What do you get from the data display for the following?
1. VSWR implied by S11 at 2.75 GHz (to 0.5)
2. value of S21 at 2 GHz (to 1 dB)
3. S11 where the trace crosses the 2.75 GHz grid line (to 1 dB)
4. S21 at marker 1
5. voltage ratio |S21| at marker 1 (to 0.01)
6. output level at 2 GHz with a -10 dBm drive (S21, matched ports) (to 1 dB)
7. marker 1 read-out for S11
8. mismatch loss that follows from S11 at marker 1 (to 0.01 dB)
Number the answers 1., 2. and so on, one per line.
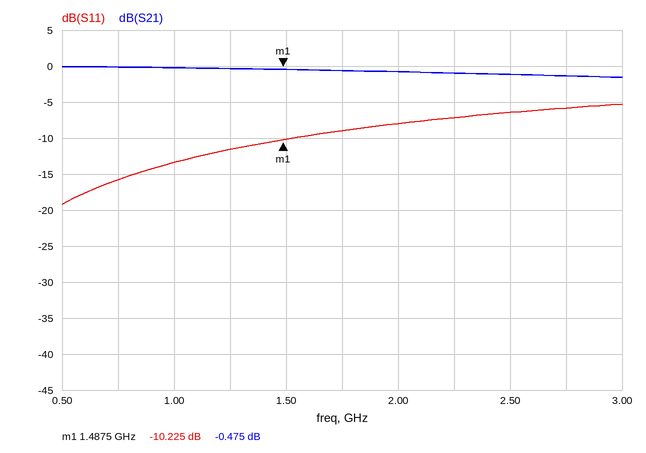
1. 3.0
2. -1 dB
3. -6 dB
4. -0.475 dB
5. 0.95
6. -11 dBm
7. -10.225 dB
8. 0.43 dB
